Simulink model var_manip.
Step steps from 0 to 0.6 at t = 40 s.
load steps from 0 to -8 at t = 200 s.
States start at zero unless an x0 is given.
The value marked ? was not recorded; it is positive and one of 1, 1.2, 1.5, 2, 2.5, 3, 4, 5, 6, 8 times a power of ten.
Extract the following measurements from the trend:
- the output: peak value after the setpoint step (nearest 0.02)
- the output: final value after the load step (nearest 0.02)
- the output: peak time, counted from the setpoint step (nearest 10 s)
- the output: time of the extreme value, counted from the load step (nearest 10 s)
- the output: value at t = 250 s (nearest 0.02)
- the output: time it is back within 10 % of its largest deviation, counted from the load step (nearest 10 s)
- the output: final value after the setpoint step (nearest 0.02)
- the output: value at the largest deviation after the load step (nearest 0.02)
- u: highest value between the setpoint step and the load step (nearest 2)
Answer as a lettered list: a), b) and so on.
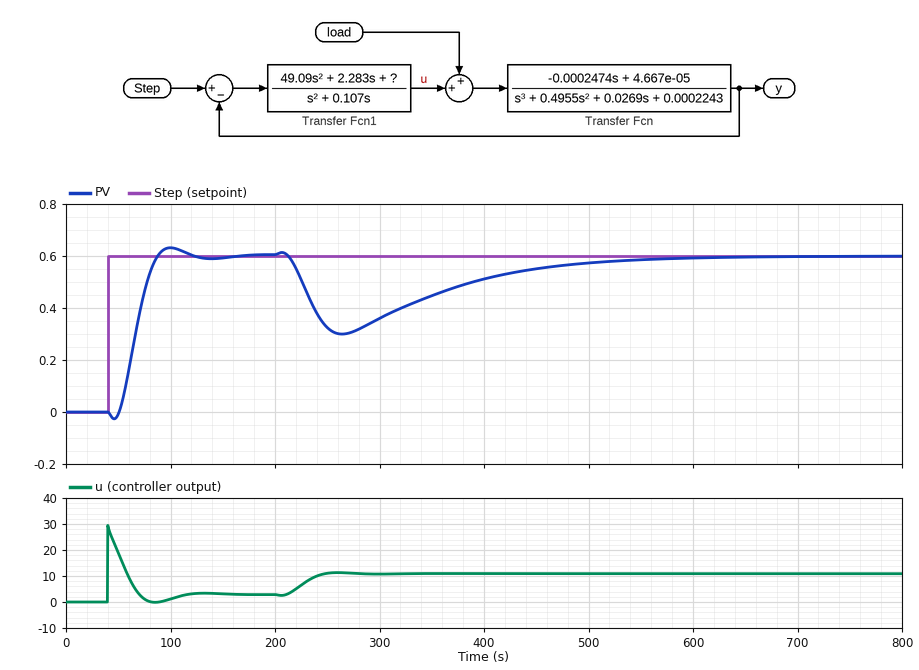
a) 0.64
b) 0.60
c) 60 s
d) 60 s
e) 0.32
f) 290 s
g) 0.60
h) 0.30
i) 30
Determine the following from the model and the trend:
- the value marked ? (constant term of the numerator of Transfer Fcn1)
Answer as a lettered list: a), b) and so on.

a) 0.02
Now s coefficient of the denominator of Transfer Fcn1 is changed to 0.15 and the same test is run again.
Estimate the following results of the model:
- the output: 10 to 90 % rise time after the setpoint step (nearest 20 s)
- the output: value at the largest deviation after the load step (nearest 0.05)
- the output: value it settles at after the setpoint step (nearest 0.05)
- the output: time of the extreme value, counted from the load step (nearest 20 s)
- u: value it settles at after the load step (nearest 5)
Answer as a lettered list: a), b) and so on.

a) 60 s
b) 0.25
c) 0.60
d) 80 s
e) 10
